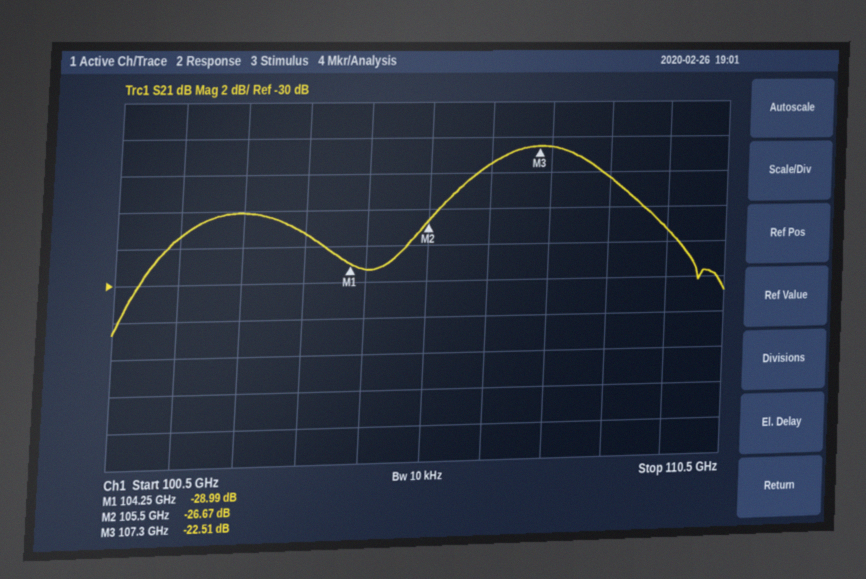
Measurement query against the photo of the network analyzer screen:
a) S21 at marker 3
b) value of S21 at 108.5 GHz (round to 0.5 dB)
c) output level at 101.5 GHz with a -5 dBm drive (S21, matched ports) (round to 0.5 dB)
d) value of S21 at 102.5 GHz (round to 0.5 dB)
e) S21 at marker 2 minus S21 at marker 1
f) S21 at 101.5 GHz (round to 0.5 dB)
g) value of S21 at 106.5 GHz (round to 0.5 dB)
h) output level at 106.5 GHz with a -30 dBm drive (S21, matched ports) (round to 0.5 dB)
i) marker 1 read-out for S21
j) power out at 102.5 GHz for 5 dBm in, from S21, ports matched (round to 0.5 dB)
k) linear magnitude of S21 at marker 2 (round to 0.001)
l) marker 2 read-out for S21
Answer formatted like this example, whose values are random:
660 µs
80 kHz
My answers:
-22.51 dB
-24.5 dB
-32.5 dBm
-26.0 dB
2.32 dB
-27.5 dB
-23.5 dB
-53.5 dBm
-28.99 dB
-21.0 dBm
0.046
-26.67 dB
